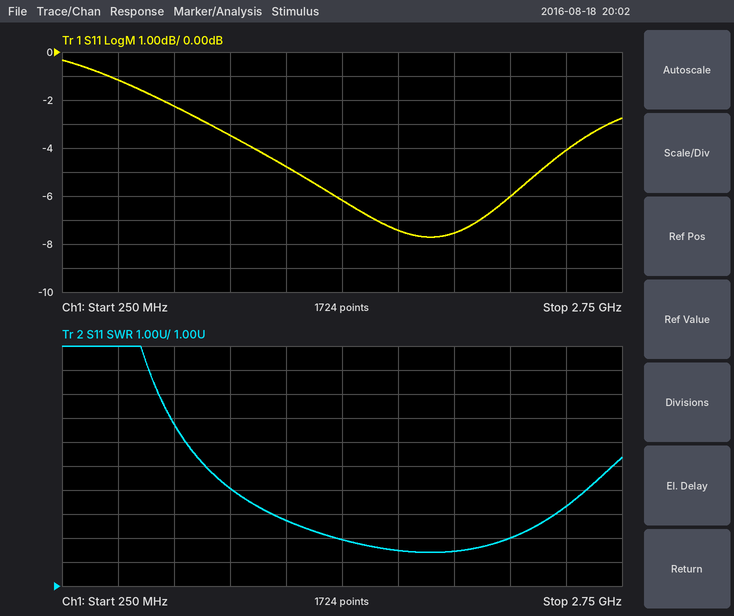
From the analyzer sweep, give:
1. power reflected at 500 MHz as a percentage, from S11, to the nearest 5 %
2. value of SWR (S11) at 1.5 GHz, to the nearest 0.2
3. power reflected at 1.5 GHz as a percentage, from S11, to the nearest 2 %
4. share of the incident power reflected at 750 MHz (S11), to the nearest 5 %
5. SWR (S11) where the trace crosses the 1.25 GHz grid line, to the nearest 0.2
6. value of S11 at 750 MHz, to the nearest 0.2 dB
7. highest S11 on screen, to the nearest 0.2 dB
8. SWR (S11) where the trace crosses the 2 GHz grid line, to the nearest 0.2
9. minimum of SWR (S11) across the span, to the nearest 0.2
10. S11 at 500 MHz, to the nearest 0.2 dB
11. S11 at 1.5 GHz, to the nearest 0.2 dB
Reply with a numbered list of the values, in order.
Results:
1. 75 %
2. 3.0
3. 24 %
4. 60 %
5. 3.8
6. -2.2 dB
7. -0.4 dB
8. 2.4
9. 2.4
10. -1.2 dB
11. -6.2 dB
